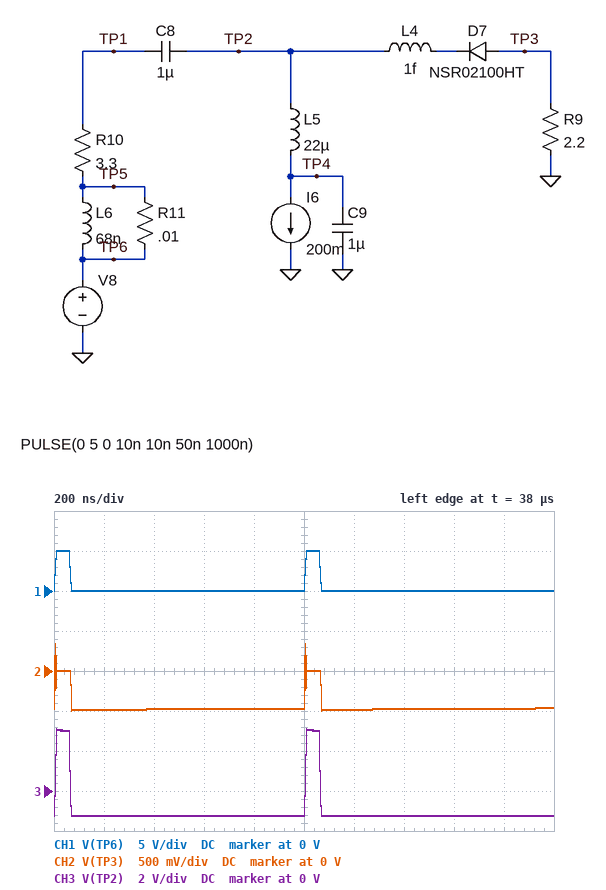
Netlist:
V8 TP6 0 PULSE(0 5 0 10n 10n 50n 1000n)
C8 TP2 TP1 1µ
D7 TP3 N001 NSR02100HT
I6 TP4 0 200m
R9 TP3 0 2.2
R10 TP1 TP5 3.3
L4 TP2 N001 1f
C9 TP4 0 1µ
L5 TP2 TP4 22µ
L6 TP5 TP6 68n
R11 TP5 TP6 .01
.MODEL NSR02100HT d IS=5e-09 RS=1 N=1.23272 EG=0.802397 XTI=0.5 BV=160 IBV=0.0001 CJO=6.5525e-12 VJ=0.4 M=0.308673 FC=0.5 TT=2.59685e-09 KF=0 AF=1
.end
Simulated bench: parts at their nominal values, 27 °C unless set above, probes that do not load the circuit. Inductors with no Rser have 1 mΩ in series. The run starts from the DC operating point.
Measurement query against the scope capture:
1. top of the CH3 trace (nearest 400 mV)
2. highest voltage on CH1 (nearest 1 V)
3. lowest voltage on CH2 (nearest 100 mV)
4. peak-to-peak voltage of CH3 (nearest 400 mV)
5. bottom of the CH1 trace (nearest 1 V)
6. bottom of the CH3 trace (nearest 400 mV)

3.2 V
5 V
-500 mV
4.4 V
0 V
-1.2 V
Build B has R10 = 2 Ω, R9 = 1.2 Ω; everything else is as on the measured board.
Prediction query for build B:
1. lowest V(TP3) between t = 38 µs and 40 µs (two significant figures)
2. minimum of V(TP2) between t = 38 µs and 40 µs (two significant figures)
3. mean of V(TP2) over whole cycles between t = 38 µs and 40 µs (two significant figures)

-280 mV
-1.1 V
-780 mV
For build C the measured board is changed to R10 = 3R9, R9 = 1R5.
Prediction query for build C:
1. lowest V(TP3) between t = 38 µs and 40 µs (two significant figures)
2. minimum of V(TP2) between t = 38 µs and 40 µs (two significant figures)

-340 mV
-1.1 V
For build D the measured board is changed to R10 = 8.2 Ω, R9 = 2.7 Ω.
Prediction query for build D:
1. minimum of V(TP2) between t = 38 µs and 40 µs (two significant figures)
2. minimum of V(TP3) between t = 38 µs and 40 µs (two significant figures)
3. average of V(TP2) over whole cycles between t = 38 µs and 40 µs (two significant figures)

-1.4 V
-590 mV
-1.2 V
